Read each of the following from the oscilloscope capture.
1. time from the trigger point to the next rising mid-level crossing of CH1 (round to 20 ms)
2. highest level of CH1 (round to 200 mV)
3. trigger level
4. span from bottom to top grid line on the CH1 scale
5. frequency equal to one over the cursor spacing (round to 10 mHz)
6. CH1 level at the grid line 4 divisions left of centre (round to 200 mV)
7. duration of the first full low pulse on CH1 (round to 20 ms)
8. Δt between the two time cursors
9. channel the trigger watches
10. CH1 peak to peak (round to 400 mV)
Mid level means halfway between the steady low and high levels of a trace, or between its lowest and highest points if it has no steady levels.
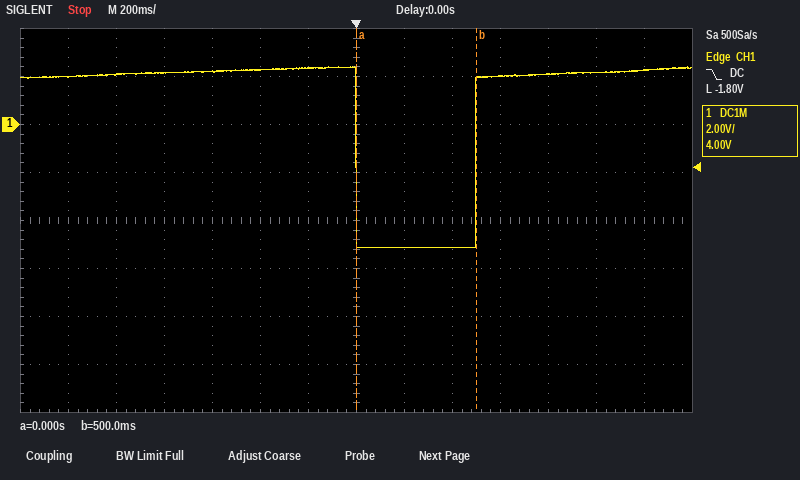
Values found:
500 ms
2.4 V
-1.80 V
16 V
2.00 Hz
2.2 V
500 ms
500 ms
CH1
7.6 V
